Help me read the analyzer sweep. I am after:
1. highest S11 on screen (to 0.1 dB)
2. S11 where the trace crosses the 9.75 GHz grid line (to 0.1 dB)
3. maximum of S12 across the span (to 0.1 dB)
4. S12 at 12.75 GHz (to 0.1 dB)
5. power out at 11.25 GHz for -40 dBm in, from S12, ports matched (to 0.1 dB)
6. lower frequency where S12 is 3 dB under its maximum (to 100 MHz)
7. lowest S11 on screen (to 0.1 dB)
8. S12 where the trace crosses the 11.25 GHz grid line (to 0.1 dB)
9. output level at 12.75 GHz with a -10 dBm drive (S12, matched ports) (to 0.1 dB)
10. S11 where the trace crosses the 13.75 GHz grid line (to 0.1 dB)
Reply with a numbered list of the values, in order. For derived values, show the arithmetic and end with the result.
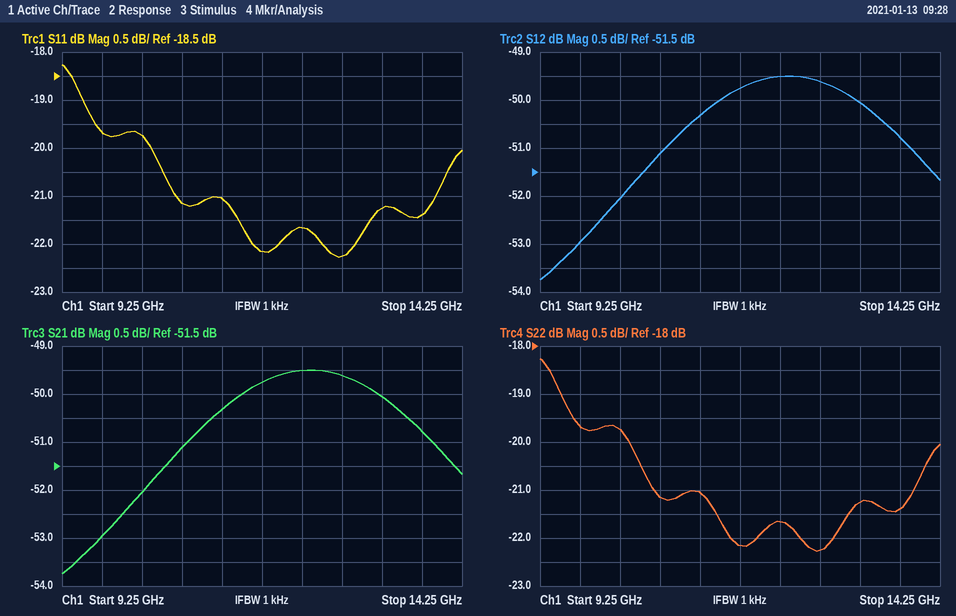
1. -18.3 dB
2. -19.7 dB
3. -49.5 dB
4. -49.6 dB
5. -40 dBm + (-50.3 dB) = -90.3 dBm
6. 10.0 GHz
7. -22.3 dB
8. -50.3 dB
9. -10 dBm + (-49.6 dB) = -59.6 dBm
10. -21.4 dB
